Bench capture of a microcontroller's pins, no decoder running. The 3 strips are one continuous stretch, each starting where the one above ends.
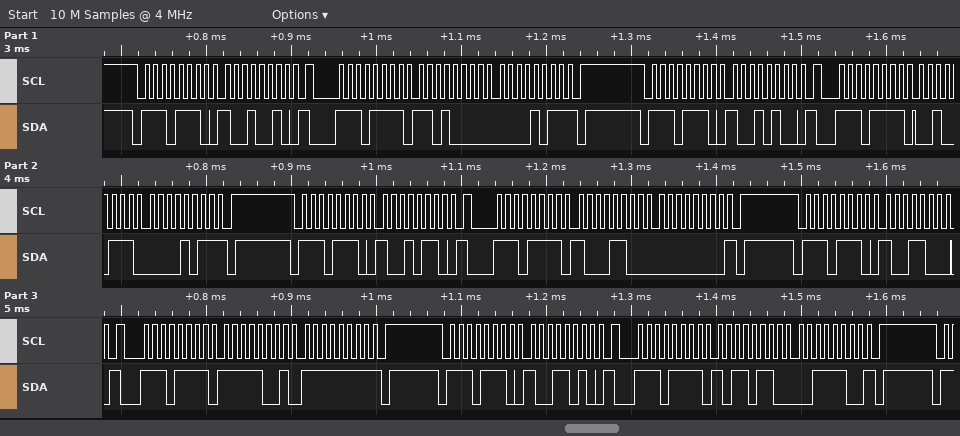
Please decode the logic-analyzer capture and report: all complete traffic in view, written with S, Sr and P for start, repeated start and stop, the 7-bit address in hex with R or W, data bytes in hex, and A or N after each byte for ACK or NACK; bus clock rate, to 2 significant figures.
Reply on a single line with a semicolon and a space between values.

S 77W A 92 A Sr 77R A D0 A 0B N P S 77W A 94 A Sr 77R A 27 A 0B N P S 77W A 96 A Sr 77R A 8C A 00 N P S 77W A 98 A Sr 77R A F9 A FF N P S 77W A 9A A Sr 77R A B6 A 3C N P; 100 kHz
